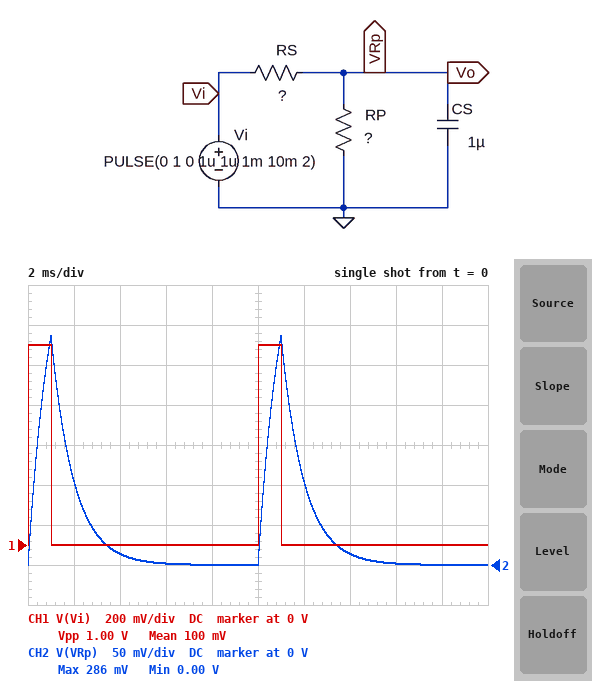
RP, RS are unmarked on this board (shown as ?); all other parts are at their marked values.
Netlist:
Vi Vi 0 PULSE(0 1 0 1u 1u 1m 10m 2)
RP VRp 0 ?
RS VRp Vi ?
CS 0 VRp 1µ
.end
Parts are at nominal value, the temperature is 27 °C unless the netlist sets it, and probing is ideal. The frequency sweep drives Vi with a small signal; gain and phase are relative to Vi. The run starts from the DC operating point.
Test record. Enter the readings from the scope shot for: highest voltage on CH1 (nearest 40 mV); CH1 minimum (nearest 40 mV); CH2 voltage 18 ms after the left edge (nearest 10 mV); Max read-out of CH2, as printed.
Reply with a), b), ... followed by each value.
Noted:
a) 1.00 V
b) 0 V
c) 0 V
d) 286 mV
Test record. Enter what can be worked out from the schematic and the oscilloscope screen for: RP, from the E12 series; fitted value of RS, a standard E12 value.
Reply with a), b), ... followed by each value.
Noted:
a) 1.8 kΩ
b) 2.2 kΩ
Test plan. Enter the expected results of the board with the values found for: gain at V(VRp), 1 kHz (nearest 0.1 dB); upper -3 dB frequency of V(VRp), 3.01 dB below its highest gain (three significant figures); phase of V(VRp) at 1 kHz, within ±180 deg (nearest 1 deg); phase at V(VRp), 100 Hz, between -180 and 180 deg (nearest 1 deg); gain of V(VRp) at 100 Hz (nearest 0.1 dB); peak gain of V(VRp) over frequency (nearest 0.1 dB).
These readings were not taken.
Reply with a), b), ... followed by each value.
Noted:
a) -22.9 dB
b) 161 Hz
c) -81 deg
d) -32 deg
e) -8.4 dB
f) -6.9 dB
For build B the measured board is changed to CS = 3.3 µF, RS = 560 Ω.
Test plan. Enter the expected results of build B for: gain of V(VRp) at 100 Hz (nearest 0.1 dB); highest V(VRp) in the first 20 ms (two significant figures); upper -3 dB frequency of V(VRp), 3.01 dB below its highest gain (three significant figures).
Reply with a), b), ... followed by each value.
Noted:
a) -4.9 dB
b) 390 mV
c) 113 Hz
